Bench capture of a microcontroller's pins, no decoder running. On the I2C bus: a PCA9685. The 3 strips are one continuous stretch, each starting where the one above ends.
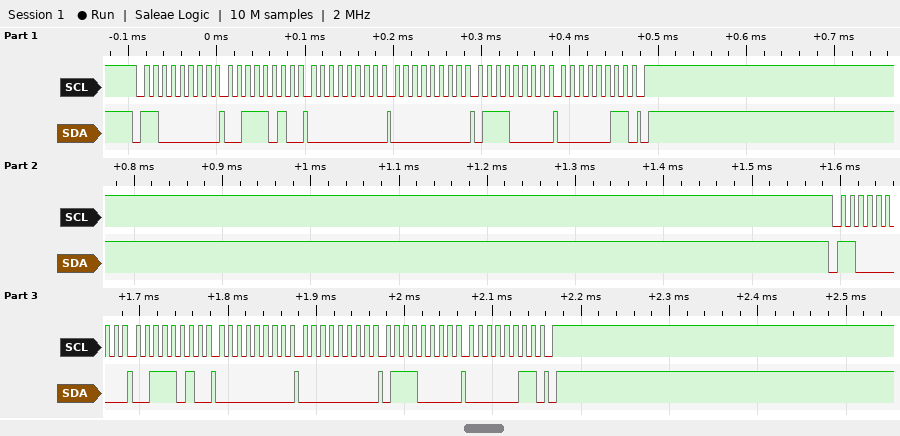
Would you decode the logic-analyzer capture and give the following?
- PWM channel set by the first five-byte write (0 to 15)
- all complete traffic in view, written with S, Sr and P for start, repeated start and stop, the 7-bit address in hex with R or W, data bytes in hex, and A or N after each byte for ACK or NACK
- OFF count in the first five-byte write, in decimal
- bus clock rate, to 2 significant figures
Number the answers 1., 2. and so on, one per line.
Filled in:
1. 13
2. S 60W A 3A A 00 A 00 A 70 A 03 A P S 60W A 3A A 00 A 00 A 70 A 03 A P
3. 880
4. 100 kHz
